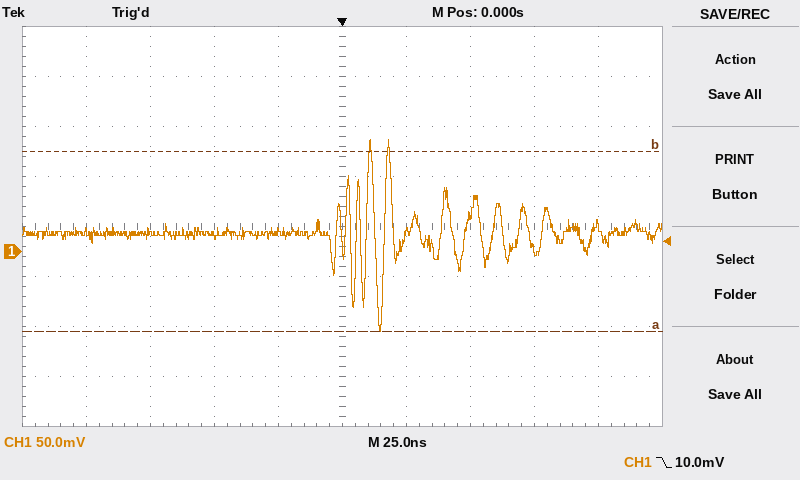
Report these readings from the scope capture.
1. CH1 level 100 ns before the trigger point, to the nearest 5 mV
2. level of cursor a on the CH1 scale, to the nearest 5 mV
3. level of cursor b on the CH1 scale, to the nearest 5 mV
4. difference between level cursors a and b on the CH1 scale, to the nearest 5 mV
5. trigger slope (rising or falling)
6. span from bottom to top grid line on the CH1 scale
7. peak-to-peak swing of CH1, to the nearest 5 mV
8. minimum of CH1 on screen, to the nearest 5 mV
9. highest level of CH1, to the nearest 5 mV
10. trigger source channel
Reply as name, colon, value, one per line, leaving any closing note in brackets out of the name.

CH1 level 100 ns before the trigger point, to the nearest 5 mV: 20 mV
level of cursor a on the CH1 scale, to the nearest 5 mV: -80 mV
level of cursor b on the CH1 scale, to the nearest 5 mV: 100 mV
difference between level cursors a and b on the CH1 scale, to the nearest 5 mV: 180 mV
trigger slope: falling
span from bottom to top grid line on the CH1 scale: 400 mV
peak-to-peak swing of CH1, to the nearest 5 mV: 190 mV
minimum of CH1 on screen, to the nearest 5 mV: -80 mV
highest level of CH1, to the nearest 5 mV: 110 mV
trigger source channel: CH1
